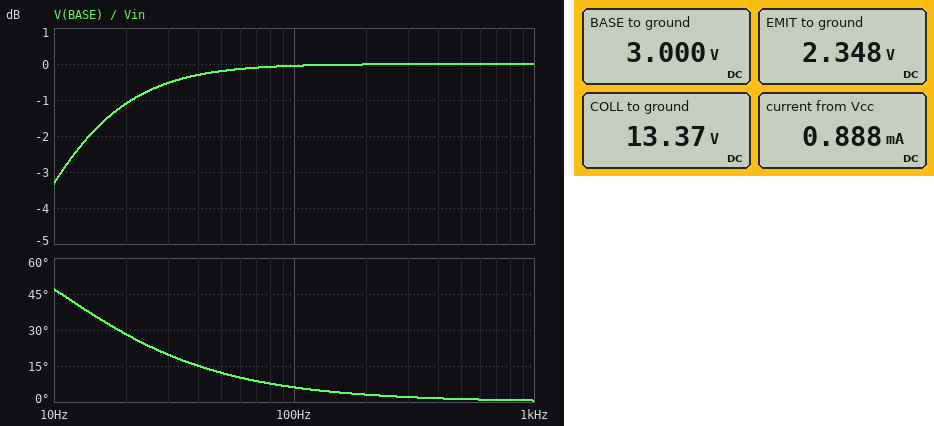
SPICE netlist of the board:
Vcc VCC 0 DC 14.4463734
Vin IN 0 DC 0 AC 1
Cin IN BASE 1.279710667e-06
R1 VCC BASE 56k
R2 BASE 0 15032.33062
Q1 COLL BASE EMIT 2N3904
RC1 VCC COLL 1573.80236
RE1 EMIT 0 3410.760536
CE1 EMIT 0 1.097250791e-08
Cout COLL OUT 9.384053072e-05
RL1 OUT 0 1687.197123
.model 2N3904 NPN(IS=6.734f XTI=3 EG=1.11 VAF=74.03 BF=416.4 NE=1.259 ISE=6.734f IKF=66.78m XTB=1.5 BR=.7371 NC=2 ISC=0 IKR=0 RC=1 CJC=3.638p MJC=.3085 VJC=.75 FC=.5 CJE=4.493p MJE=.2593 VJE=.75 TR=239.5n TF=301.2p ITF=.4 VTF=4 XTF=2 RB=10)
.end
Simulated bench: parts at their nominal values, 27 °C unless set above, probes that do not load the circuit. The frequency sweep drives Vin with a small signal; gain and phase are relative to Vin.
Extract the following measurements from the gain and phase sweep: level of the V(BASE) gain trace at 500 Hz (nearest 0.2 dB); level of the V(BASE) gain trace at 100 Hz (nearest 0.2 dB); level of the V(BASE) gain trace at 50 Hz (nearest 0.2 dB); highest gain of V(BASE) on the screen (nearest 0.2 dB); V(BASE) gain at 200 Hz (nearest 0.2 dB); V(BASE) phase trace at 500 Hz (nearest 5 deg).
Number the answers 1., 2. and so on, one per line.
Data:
1. 0 dB
2. 0 dB
3. -0.2 dB
4. 0 dB
5. 0 dB
6. 0 deg
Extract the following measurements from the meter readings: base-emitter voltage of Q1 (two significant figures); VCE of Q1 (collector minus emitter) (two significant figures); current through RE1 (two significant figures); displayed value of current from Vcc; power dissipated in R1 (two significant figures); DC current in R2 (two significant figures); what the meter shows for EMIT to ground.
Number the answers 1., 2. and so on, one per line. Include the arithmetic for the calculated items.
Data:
1. 3 V - 2.348 V = 650 mV
2. 13.37 V - 2.348 V = 11 V
3. (2.348 V) / 3.411 kΩ = 690 µA
4. 0.888 mA
5. (14.45 V - 3 V)^2 / 56 kΩ = 2.3 mW
6. (3 V) / 15.03 kΩ = 200 µA
7. 2.348 V
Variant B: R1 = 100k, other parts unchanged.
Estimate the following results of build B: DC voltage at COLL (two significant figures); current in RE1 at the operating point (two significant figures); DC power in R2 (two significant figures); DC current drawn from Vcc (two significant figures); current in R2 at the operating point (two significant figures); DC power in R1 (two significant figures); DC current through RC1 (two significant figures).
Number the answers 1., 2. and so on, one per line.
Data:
1. 14 V
2. 360 µA
3. 230 µW
4. 480 µA
5. 120 µA
6. 1.6 mW
7. 350 µA
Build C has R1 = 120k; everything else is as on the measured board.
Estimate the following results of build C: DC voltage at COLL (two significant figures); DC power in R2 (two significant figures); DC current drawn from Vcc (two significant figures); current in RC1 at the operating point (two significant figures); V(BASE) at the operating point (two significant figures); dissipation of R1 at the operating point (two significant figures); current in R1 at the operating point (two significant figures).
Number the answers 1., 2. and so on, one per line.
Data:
1. 14 V
2. 170 µW
3. 380 µA
4. 280 µA
5. 1.6 V
6. 1.4 mW
7. 110 µA
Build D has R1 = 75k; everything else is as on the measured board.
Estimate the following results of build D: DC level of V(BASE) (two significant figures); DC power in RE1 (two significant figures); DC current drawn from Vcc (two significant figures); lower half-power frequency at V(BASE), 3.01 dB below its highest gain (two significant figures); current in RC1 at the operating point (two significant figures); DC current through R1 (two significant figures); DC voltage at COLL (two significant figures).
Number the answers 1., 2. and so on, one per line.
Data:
1. 2.4 V
2. 870 µW
3. 660 µA
4. 10 Hz
5. 500 µA
6. 160 µA
7. 14 V
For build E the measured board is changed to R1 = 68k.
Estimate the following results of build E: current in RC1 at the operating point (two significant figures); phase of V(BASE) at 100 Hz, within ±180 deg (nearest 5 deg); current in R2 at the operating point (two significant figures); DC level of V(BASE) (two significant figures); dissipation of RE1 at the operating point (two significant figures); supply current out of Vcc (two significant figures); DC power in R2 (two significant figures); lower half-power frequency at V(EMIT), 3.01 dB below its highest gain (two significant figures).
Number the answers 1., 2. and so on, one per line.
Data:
1. 560 µA
2. 5 deg
3. 170 µA
4. 2.6 V
5. 1.1 mW
6. 730 µA
7. 440 µW
8. 10 Hz
